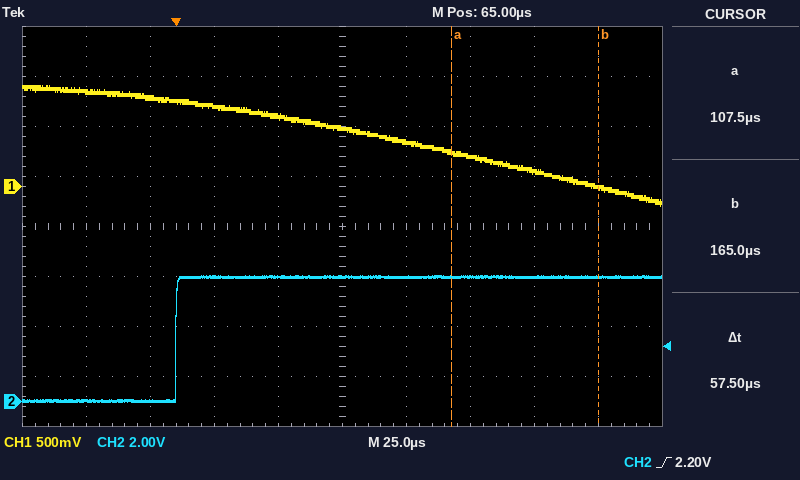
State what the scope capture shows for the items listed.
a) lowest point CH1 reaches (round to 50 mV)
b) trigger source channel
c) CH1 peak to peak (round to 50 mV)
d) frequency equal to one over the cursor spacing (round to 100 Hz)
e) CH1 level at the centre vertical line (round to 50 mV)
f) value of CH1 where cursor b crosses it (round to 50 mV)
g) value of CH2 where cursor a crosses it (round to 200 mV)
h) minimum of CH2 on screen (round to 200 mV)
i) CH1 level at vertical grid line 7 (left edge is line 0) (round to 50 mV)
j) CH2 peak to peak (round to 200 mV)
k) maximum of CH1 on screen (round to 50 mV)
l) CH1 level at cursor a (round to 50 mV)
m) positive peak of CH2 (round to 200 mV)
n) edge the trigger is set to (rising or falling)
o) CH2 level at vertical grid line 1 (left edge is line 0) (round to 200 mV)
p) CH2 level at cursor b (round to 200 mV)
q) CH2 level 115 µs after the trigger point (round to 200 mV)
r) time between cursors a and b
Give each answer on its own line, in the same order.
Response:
-200 mV
CH2
1.20 V
17.4 kHz
600 mV
0 mV
5.0 V
0.0 V
300 mV
5.0 V
1.00 V
350 mV
5.0 V
rising
0.0 V
5.0 V
5.0 V
57.5 µs
